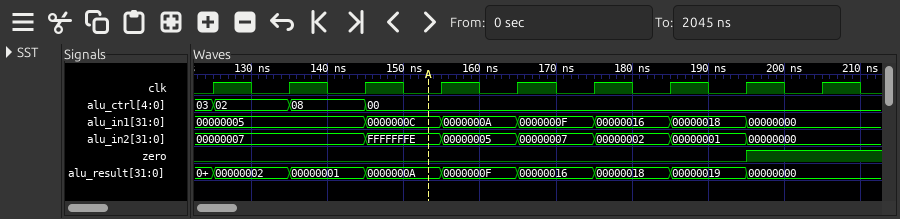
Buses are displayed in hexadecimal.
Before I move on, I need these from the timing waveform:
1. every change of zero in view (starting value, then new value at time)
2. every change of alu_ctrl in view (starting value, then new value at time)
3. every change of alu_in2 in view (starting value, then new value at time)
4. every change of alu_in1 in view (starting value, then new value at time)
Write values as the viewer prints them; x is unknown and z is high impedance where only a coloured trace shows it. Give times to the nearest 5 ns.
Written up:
0, 1 at 195 ns
03, 02 at 125 ns, 08 at 135 ns, 00 at 145 ns
00000007, FFFFFFFE at 145 ns, 00000005 at 155 ns, 00000007 at 165 ns, 00000002 at 175 ns, 00000001 at 185 ns, 00000000 at 195 ns
00000005, 0000000C at 145 ns, 0000000A at 155 ns, 0000000F at 165 ns, 00000016 at 175 ns, 00000018 at 185 ns, 00000000 at 195 ns
